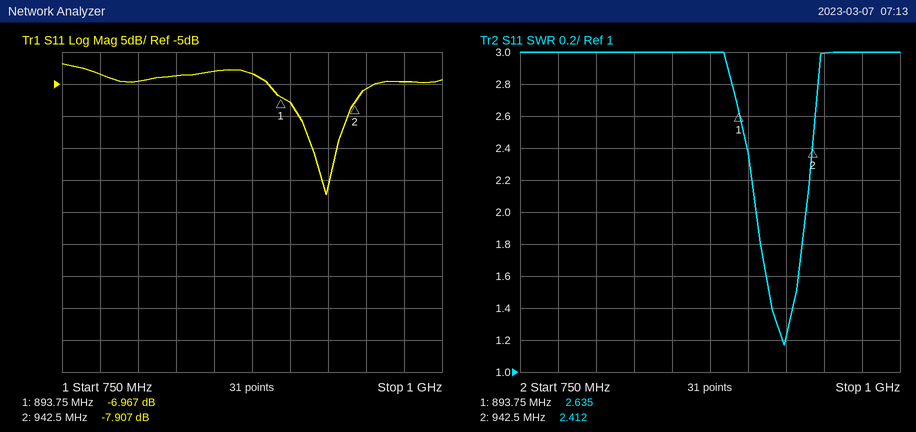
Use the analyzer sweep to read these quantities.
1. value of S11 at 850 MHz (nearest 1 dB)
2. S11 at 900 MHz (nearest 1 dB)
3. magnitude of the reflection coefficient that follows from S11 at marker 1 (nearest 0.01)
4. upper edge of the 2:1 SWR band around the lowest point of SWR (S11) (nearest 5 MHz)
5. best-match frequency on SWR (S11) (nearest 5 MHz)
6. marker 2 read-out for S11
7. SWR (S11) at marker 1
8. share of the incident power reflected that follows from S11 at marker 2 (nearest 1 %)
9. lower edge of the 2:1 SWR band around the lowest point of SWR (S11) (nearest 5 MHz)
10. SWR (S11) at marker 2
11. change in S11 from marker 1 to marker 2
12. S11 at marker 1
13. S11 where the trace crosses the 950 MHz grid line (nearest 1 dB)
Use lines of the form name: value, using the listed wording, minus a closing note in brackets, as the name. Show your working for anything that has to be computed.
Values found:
value of S11 at 850 MHz: -3 dB
S11 at 900 MHz: -8 dB
magnitude of the reflection coefficient that follows from S11 at marker 1: 10^(-6.967/20) ≈ 0.45
upper edge of the 2:1 SWR band around the lowest point of SWR (S11): 940 MHz
best-match frequency on SWR (S11): 925 MHz
marker 2 read-out for S11: -7.907 dB
SWR (S11) at marker 1: 2.635
share of the incident power reflected that follows from S11 at marker 2: 10^(-7.907/10) ≈ 16 %
lower edge of the 2:1 SWR band around the lowest point of SWR (S11): 905 MHz
SWR (S11) at marker 2: 2.412
change in S11 from marker 1 to marker 2: -7.907 − (-6.967) = -0.940 dB
S11 at marker 1: -6.967 dB
S11 where the trace crosses the 950 MHz grid line: -6 dB
